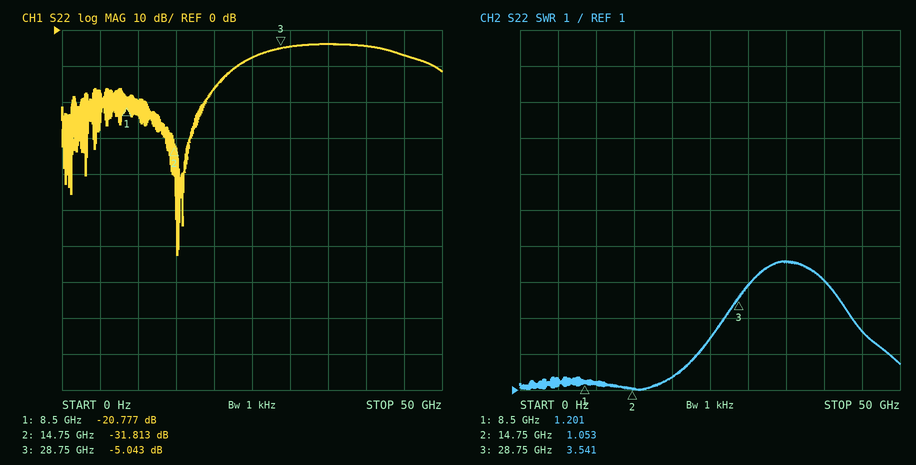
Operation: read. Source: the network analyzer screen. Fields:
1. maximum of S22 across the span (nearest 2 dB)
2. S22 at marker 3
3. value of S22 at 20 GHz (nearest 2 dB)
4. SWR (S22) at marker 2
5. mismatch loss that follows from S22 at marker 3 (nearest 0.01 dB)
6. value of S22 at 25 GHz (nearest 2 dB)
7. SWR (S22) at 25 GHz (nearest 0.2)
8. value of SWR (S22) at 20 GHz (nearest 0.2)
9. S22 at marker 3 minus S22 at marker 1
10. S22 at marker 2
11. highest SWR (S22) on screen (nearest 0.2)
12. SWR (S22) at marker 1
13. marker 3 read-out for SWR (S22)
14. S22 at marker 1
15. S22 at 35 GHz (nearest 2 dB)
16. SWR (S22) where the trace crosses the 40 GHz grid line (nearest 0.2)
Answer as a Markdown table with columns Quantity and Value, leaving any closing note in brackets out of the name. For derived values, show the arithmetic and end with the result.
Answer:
| Quantity | Value |
|---|---|
| maximum of S22 across the span | -4 dB |
| S22 at marker 3 | -5.043 dB |
| value of S22 at 20 GHz | -16 dB |
| SWR (S22) at marker 2 | 1.053 |
| mismatch loss that follows from S22 at marker 3 | −10 log10(1 − 10^(-5.043/10)) ≈ 1.63 dB |
| value of S22 at 25 GHz | -8 dB |
| SWR (S22) at 25 GHz | 2.4 |
| value of SWR (S22) at 20 GHz | 1.4 |
| S22 at marker 3 minus S22 at marker 1 | -5.043 − (-20.777) = 15.734 dB |
| S22 at marker 2 | -31.813 dB |
| highest SWR (S22) on screen | 4.6 |
| SWR (S22) at marker 1 | 1.201 |
| marker 3 read-out for SWR | 3.541 |
| S22 at marker 1 | -20.777 dB |
| S22 at 35 GHz | -4 dB |
| SWR (S22) where the trace crosses the 40 GHz grid line | 4.0 |
